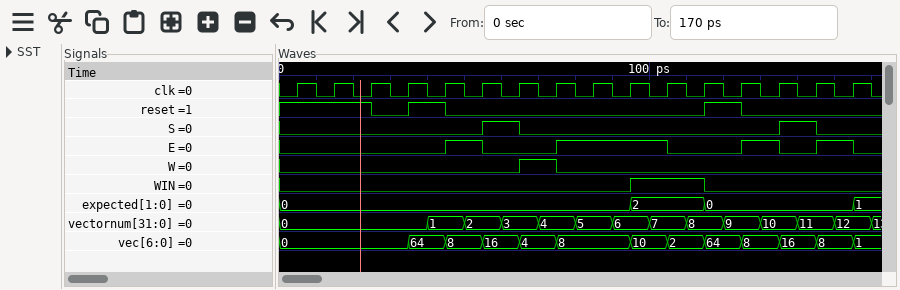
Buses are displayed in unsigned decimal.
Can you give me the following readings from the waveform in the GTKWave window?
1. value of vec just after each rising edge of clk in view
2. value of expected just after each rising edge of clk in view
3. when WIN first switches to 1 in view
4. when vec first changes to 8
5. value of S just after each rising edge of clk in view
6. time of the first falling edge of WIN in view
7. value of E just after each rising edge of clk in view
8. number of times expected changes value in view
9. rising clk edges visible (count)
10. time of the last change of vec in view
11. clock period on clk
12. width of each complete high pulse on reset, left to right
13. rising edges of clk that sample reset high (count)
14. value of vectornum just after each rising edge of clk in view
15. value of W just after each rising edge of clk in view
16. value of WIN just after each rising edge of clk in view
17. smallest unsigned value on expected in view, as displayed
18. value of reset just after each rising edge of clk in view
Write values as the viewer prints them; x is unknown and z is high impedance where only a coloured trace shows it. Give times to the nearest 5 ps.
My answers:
0, 0, 0, 64, 8, 16, 4, 8, 8, 10, 2, 64, 8, 16, 8, 1
0, 0, 0, 0, 0, 0, 0, 0, 0, 2, 2, 0, 0, 0, 0, 1
95 ps
45 ps
0 0 0 0 0 1 0 0 0 0 0 0 0 1 0 0
115 ps
0 0 0 0 1 0 0 1 1 1 0 0 1 0 1 0
3
16
155 ps
10 ps
10 ps, 10 ps
5
0, 0, 0, 0, 1, 2, 3, 4, 5, 6, 7, 8, 9, 10, 11, 12
0 0 0 0 0 0 1 0 0 0 0 0 0 0 0 0
0 0 0 0 0 0 0 0 0 1 1 0 0 0 0 0
0
1 1 0 1 0 0 0 0 0 0 0 1 0 0 0 0
